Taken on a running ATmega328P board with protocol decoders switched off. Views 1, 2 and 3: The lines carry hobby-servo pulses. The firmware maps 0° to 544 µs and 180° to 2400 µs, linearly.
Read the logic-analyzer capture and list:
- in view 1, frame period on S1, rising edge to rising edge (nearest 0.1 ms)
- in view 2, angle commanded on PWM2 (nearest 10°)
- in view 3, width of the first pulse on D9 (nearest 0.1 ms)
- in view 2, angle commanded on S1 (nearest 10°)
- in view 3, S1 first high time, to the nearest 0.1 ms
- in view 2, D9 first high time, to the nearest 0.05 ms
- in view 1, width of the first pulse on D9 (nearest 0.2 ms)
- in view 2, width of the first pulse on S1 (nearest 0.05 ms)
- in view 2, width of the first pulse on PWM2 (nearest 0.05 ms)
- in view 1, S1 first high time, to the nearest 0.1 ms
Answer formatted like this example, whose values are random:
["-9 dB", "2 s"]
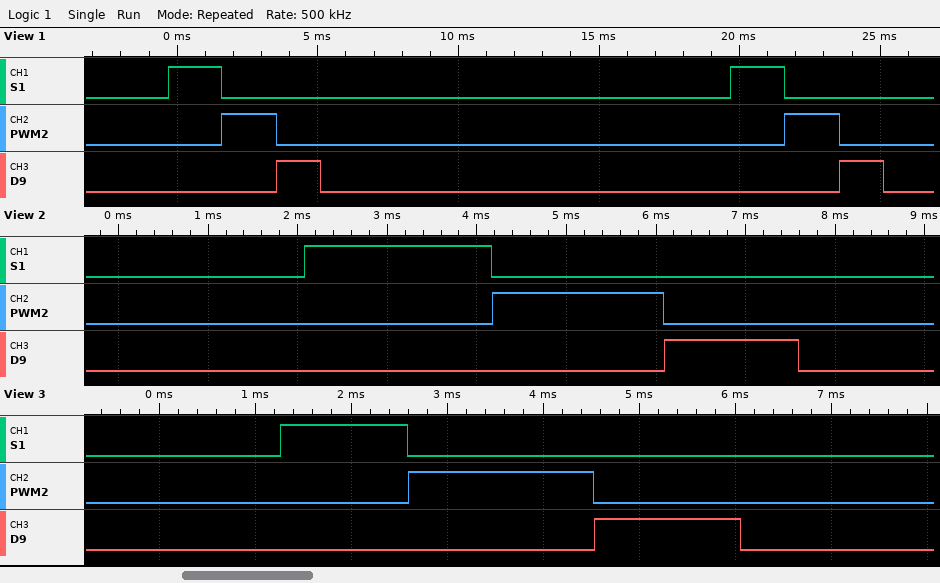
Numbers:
["20.0 ms", "130°", "1.5 ms", "150°", "1.3 ms", "1.50 ms", "1.6 ms", "2.10 ms", "1.90 ms", "1.9 ms"]
